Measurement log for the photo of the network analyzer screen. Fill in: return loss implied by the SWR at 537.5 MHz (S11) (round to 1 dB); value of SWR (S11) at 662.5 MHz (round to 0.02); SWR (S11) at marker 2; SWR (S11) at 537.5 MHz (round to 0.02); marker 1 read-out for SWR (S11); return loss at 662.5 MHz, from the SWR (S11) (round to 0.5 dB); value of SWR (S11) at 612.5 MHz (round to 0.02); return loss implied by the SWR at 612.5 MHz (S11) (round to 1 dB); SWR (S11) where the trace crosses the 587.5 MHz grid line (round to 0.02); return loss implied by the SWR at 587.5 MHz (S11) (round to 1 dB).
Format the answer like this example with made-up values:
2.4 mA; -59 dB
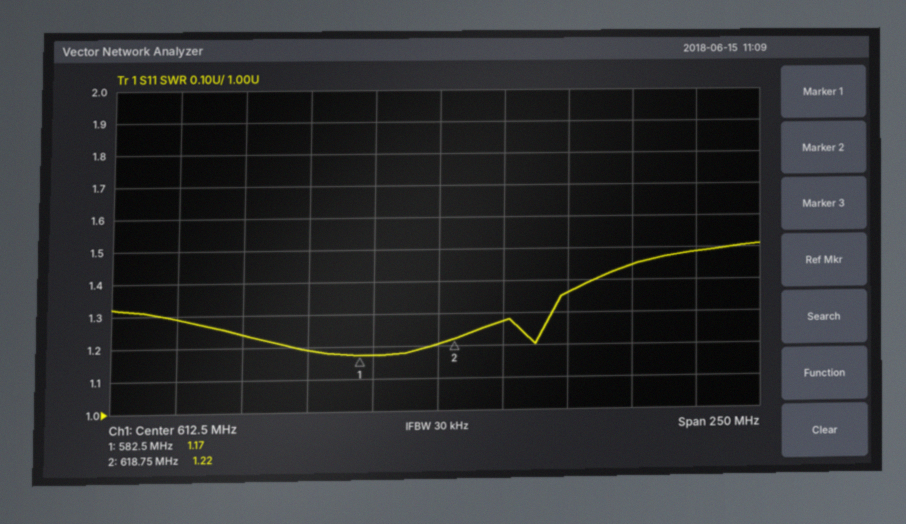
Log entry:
19 dB; 1.36; 1.22; 1.24; 1.17; 16.5 dB; 1.20; 21 dB; 1.18; 22 dB
